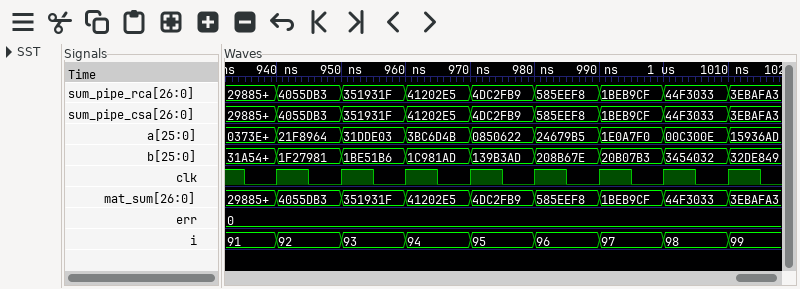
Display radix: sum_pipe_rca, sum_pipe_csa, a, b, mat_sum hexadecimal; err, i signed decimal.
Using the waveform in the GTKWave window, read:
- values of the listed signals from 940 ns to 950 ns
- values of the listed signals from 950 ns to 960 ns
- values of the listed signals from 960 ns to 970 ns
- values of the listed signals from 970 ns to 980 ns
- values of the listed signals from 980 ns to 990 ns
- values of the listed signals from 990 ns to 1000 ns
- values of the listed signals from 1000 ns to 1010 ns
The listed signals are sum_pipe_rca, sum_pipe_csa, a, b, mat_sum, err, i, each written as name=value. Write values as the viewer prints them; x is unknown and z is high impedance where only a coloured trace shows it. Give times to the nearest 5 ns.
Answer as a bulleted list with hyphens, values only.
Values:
- sum_pipe_rca=4055DB3, sum_pipe_csa=4055DB3, a=21F8964, b=1F27981, mat_sum=4055DB3, err=0, i=92
- sum_pipe_rca=351931F, sum_pipe_csa=351931F, a=31DDE03, b=1BE51B6, mat_sum=351931F, err=0, i=93
- sum_pipe_rca=41202E5, sum_pipe_csa=41202E5, a=3BC6D4B, b=1C981AD, mat_sum=41202E5, err=0, i=94
- sum_pipe_rca=4DC2FB9, sum_pipe_csa=4DC2FB9, a=0850622, b=139B3AD, mat_sum=4DC2FB9, err=0, i=95
- sum_pipe_rca=585EEF8, sum_pipe_csa=585EEF8, a=24679B5, b=208B67E, mat_sum=585EEF8, err=0, i=96
- sum_pipe_rca=1BEB9CF, sum_pipe_csa=1BEB9CF, a=1E0A7F0, b=20B07B3, mat_sum=1BEB9CF, err=0, i=97
- sum_pipe_rca=44F3033, sum_pipe_csa=44F3033, a=00C300E, b=3454032, mat_sum=44F3033, err=0, i=98
